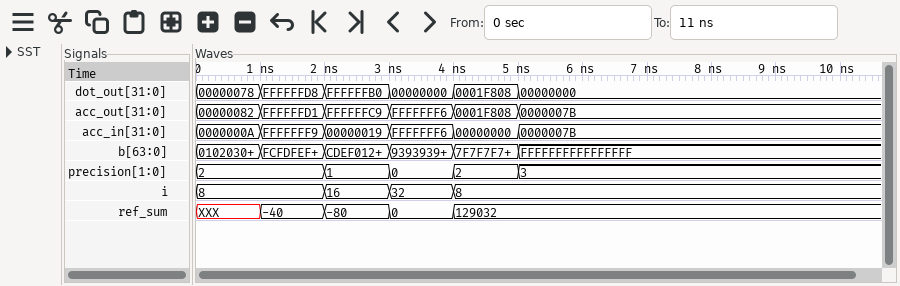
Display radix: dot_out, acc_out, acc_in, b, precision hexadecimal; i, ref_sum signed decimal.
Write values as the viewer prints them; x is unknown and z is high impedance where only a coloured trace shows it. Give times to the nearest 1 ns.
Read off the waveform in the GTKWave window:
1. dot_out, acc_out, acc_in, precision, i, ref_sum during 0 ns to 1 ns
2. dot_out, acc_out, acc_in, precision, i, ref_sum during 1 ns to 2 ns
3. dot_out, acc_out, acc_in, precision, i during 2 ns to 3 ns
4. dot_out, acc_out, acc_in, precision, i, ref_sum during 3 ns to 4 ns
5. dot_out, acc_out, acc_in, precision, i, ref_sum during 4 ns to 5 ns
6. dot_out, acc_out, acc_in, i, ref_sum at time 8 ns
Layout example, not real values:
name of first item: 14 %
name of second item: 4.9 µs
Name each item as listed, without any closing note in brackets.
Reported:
dot_out, acc_out, acc_in, precision, i, ref_sum during 0 ns to 1 ns: dot_out=00000078, acc_out=00000082, acc_in=0000000A, precision=2, i=8, ref_sum=XXX
dot_out, acc_out, acc_in, precision, i, ref_sum during 1 ns to 2 ns: dot_out=FFFFFFD8, acc_out=FFFFFFD1, acc_in=FFFFFFF9, precision=2, i=8, ref_sum=-40
dot_out, acc_out, acc_in, precision, i during 2 ns to 3 ns: dot_out=FFFFFFB0, acc_out=FFFFFFC9, acc_in=00000019, precision=1, i=16
dot_out, acc_out, acc_in, precision, i, ref_sum during 3 ns to 4 ns: dot_out=00000000, acc_out=FFFFFFF6, acc_in=FFFFFFF6, precision=0, i=32, ref_sum=0
dot_out, acc_out, acc_in, precision, i, ref_sum during 4 ns to 5 ns: dot_out=0001F808, acc_out=0001F808, acc_in=00000000, precision=2, i=8, ref_sum=129032
dot_out, acc_out, acc_in, i, ref_sum at time 8 ns: dot_out=00000000, acc_out=0000007B, acc_in=0000007B, i=8, ref_sum=129032
